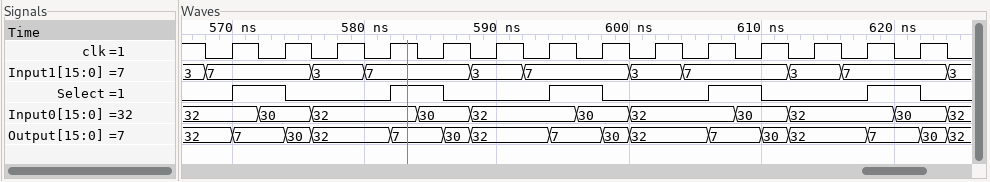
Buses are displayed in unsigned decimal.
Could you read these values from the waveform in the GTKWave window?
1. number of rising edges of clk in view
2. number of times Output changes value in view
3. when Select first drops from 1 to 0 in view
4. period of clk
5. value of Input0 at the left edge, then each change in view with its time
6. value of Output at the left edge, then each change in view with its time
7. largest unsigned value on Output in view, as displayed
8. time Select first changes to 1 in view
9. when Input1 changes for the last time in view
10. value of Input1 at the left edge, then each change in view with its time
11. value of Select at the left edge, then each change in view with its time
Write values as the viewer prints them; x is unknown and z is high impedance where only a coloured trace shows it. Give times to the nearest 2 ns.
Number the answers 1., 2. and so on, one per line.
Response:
1. 14
2. 15
3. 574 ns
4. 4 ns
5. 32, 30 at 572 ns, 32 at 576 ns, 30 at 584 ns, 32 at 588 ns, 30 at 596 ns, 32 at 600 ns, 30 at 608 ns, 32 at 612 ns, 30 at 620 ns, 32 at 624 ns
6. 32, 7 at 570 ns, 30 at 574 ns, 32 at 576 ns, 7 at 582 ns, 30 at 586 ns, 32 at 588 ns, 7 at 594 ns, 30 at 598 ns, 32 at 600 ns, 7 at 606 ns, 30 at 610 ns, 32 at 612 ns, 7 at 618 ns, 30 at 622 ns, 32 at 624 ns
7. 32
8. 570 ns
9. 624 ns
10. 3, 7 at 568 ns, 3 at 576 ns, 7 at 580 ns, 3 at 588 ns, 7 at 592 ns, 3 at 600 ns, 7 at 604 ns, 3 at 612 ns, 7 at 616 ns, 3 at 624 ns
11. 0, 1 at 570 ns, 0 at 574 ns, 1 at 582 ns, 0 at 586 ns, 1 at 594 ns, 0 at 598 ns, 1 at 606 ns, 0 at 610 ns, 1 at 618 ns, 0 at 622 ns
